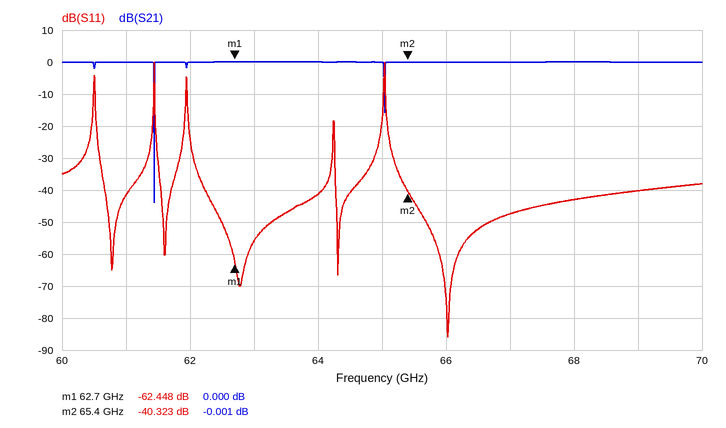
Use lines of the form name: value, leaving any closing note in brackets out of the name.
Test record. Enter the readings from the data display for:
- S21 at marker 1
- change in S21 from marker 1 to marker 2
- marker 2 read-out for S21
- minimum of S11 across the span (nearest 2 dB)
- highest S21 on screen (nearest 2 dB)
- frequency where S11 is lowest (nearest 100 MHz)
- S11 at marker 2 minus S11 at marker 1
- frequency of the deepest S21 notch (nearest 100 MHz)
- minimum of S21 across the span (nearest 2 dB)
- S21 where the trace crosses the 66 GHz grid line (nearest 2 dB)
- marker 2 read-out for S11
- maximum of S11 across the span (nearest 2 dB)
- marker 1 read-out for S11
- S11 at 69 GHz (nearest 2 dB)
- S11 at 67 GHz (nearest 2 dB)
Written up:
S21 at marker 1: 0.000 dB
change in S21 from marker 1 to marker 2: -0.001 dB
marker 2 read-out for S21: -0.001 dB
minimum of S11 across the span: -86 dB
highest S21 on screen: 0 dB
frequency where S11 is lowest: 66.0 GHz
S11 at marker 2 minus S11 at marker 1: 22.125 dB
frequency of the deepest S21 notch: 61.4 GHz
minimum of S21 across the span: -44 dB
S21 where the trace crosses the 66 GHz grid line: 0 dB
marker 2 read-out for S11: -40.323 dB
maximum of S11 across the span: 0 dB
marker 1 read-out for S11: -62.448 dB
S11 at 69 GHz: -40 dB
S11 at 67 GHz: -48 dB
